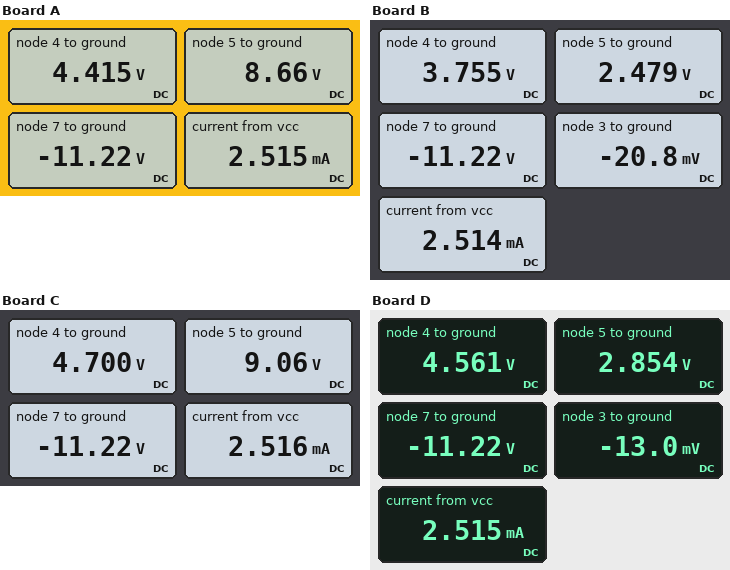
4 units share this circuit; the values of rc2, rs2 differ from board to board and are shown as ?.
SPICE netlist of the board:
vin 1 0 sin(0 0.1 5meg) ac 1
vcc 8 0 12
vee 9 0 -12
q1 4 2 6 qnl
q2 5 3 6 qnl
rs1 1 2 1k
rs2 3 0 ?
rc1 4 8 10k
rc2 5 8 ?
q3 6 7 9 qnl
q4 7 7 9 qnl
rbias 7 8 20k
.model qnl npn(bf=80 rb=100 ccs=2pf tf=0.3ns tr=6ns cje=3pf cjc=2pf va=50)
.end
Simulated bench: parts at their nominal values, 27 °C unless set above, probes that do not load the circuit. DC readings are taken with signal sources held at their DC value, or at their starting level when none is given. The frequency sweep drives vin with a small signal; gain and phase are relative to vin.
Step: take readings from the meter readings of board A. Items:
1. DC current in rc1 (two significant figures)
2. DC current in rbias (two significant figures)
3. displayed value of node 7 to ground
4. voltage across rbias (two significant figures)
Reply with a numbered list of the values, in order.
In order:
1. 760 µA
2. 1.2 mA
3. -11.22 V
4. 23 V
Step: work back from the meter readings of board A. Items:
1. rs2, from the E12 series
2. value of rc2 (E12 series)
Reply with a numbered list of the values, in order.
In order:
1. 2.7 kΩ
2. 5.6 kΩ
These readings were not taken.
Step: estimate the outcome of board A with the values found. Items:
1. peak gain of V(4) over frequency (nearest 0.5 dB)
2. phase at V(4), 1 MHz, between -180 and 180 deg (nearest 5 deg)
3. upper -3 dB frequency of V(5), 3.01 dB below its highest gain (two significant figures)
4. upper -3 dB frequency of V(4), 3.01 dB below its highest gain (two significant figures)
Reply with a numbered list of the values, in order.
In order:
1. 37.5 dB
2. 120 deg
3. 700 kHz
4. 690 kHz
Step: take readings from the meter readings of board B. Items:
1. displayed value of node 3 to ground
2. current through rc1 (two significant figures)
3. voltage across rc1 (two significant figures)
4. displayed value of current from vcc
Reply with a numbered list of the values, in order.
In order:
1. -20.8 mV
2. 820 µA
3. 8.2 V
4. 2.514 mA
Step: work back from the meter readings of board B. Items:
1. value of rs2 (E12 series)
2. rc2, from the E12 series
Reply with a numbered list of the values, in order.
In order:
1. 3.3 kΩ
2. 18 kΩ
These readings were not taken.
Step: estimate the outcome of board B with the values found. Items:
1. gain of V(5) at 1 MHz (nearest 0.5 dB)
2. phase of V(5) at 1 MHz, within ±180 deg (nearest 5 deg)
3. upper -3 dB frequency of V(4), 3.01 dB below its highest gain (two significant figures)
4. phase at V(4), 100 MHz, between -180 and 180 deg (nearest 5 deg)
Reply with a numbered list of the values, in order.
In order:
1. 29.0 dB
2. -75 deg
3. 260 kHz
4. 60 deg
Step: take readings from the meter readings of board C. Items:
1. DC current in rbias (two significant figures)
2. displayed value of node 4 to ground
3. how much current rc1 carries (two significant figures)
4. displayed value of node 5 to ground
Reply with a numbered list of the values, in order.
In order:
1. 1.2 mA
2. 4.700 V
3. 730 µA
4. 9.06 V
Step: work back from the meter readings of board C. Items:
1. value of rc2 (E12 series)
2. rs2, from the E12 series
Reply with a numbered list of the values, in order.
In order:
1. 4.7 kΩ
2. 2.2 kΩ
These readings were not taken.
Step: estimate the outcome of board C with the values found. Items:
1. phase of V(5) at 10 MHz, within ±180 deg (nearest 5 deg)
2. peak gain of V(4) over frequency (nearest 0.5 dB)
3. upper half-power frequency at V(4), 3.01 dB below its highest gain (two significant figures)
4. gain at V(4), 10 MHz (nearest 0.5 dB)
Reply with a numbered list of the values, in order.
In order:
1. -85 deg
2. 38.0 dB
3. 780 kHz
4. 13.5 dB
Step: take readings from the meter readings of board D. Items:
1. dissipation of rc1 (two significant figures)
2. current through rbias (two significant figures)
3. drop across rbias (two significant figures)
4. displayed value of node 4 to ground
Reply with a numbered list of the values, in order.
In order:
1. 5.5 mW
2. 1.2 mA
3. 23 V
4. 4.561 V
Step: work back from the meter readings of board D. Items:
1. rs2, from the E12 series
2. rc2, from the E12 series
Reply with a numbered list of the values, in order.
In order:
1. 1.8 kΩ
2. 15 kΩ
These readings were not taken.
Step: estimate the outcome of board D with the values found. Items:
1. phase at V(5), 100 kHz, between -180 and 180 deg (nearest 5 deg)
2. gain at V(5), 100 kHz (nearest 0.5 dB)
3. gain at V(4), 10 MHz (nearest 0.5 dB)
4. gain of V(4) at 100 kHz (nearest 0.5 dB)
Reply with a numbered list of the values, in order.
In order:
1. -15 deg
2. 41.0 dB
3. 12.5 dB
4. 37.5 dB
